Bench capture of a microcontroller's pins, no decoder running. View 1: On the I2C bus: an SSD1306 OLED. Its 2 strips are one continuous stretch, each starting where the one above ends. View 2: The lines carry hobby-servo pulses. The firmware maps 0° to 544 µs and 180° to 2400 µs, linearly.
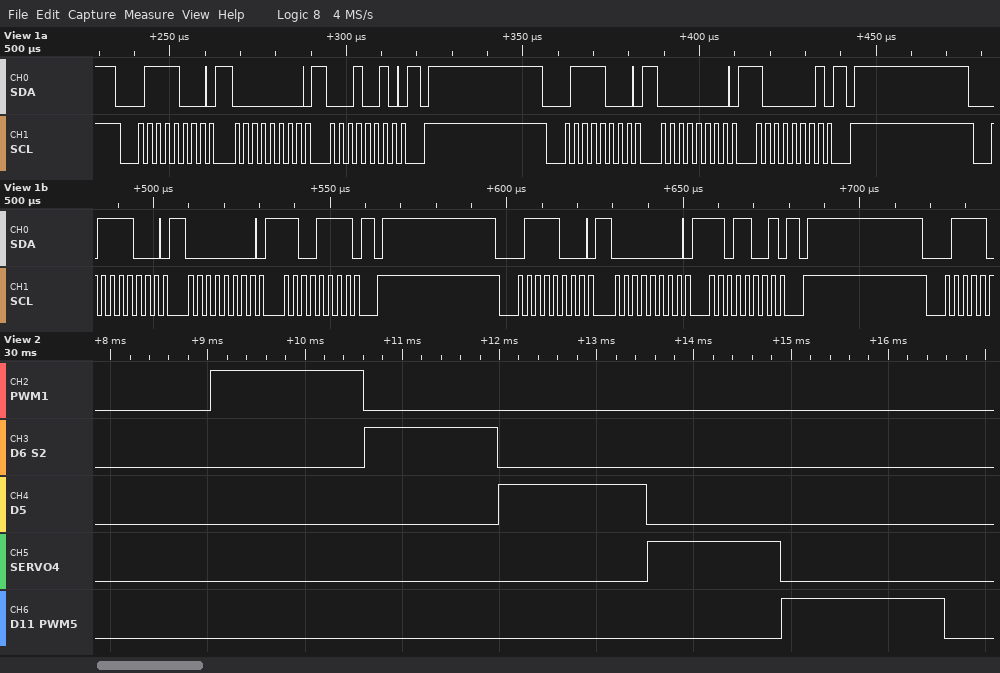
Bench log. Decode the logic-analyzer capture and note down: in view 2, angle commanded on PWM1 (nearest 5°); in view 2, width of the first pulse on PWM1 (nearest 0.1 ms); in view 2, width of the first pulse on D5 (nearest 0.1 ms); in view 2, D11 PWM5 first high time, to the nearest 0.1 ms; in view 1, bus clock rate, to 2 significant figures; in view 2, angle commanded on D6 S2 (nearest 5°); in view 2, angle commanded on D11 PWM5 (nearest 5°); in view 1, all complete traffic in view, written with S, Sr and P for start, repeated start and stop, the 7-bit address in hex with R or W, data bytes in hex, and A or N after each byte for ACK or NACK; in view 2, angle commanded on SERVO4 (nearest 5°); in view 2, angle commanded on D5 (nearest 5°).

100°
1.6 ms
1.5 ms
1.7 ms
400 kHz
80°
110°
S 3CW A 00 A 12 A P S 3CW A 00 A 81 A P S 3CW A 00 A CF A P S 3CW A 00 A D9 A P
80°
95°
